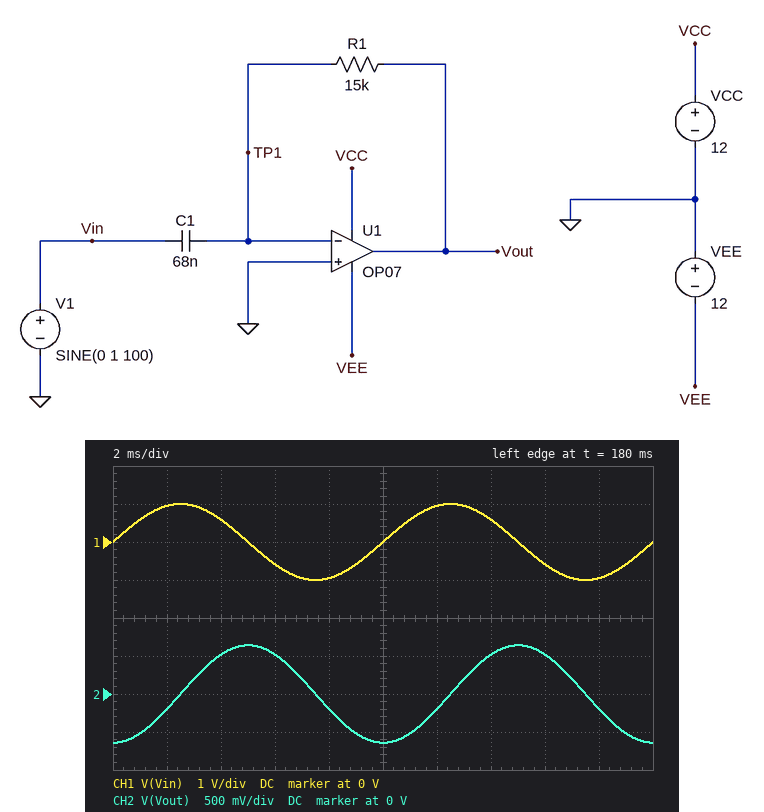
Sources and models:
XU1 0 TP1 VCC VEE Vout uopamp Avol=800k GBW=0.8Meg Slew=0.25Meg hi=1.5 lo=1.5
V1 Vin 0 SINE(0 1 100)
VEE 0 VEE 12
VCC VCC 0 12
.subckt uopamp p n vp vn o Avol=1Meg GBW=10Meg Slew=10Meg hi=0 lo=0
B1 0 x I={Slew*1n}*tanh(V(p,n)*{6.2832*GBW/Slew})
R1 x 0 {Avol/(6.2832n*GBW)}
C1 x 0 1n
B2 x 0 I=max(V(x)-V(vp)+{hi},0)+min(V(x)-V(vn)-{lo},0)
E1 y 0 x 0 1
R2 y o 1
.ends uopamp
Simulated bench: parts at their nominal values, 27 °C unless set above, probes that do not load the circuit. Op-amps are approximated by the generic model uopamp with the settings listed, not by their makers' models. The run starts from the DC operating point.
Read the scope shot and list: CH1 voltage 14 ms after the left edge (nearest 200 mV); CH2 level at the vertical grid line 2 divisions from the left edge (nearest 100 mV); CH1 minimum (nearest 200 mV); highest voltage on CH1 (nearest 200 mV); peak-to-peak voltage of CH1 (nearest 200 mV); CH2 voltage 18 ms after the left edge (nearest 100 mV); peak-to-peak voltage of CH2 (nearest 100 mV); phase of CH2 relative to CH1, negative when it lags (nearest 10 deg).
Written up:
600 mV
500 mV
-1.0 V
1.0 V
2.0 V
-200 mV
1.3 V
-90 deg
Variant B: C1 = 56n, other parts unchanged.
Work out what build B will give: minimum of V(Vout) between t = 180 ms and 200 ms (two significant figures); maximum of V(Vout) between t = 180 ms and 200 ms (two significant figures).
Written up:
-530 mV
530 mV
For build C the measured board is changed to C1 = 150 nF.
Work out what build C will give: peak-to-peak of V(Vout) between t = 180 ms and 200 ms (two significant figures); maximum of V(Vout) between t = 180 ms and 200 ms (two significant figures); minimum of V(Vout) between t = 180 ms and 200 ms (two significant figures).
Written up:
2.8 V
1.4 V
-1.4 V
